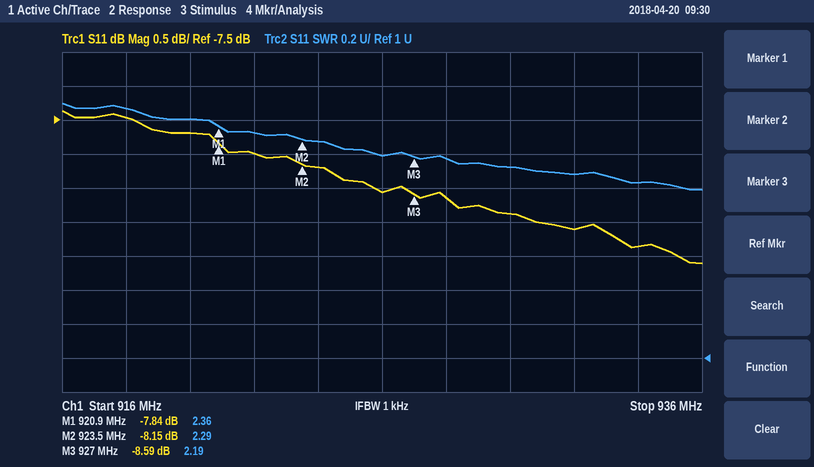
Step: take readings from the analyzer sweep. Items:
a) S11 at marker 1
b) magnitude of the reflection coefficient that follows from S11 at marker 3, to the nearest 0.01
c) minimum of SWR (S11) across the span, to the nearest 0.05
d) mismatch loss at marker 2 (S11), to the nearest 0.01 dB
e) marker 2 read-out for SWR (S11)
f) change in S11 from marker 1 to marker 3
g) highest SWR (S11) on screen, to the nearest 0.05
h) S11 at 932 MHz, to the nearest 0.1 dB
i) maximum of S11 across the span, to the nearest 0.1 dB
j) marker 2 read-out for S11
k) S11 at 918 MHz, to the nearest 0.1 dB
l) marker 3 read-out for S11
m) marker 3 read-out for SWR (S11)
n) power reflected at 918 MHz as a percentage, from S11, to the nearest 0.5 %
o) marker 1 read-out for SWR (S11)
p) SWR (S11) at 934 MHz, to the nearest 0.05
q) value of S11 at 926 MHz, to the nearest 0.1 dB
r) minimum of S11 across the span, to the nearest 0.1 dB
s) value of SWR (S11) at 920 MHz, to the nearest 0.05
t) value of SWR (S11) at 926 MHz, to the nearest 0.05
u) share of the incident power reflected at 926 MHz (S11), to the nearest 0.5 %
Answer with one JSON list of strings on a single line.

["-7.84 dB", "0.37", "2.00", "0.72 dB", "2.29", "-0.75 dB", "2.50", "-9.1 dB", "-7.4 dB", "-8.15 dB", "-7.5 dB", "-8.59 dB", "2.19", "18.0 %", "2.36", "2.05", "-8.6 dB", "-9.6 dB", "2.40", "2.20", "14.0 %"]
